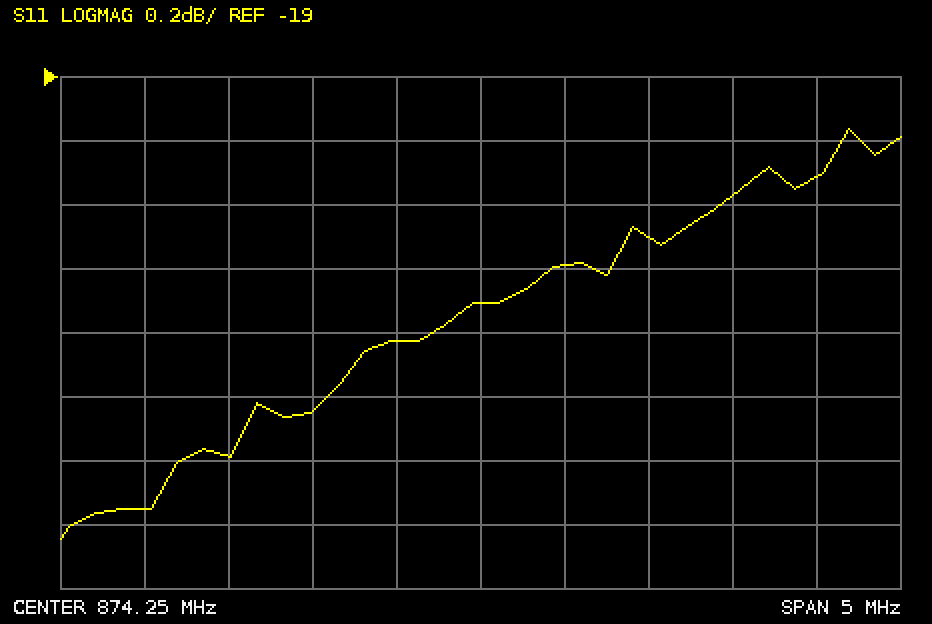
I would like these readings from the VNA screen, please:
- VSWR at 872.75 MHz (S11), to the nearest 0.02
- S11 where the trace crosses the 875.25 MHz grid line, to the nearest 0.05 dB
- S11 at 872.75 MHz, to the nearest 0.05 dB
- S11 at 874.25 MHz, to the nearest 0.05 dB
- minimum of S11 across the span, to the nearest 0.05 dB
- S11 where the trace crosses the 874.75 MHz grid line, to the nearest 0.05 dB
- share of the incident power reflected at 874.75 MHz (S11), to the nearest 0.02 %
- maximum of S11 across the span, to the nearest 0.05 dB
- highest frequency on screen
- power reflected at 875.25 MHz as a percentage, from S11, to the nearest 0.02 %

1.22
-19.50 dB
-20.20 dB
-19.70 dB
-20.45 dB
-19.60 dB
1.10 %
-19.15 dB
876.75 MHz
1.12 %
